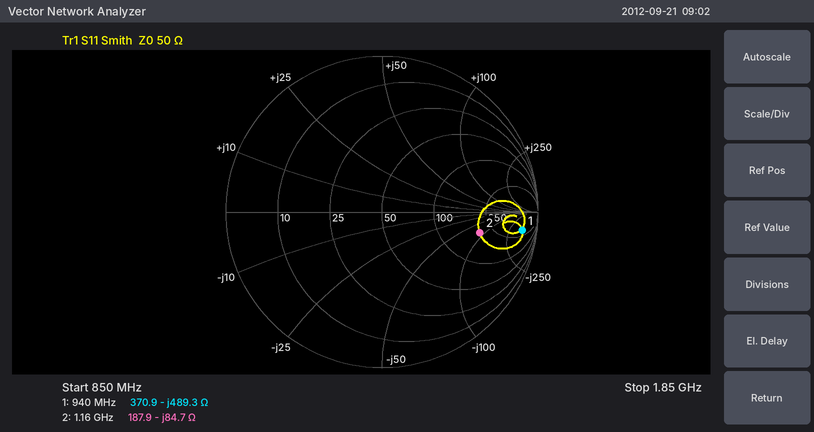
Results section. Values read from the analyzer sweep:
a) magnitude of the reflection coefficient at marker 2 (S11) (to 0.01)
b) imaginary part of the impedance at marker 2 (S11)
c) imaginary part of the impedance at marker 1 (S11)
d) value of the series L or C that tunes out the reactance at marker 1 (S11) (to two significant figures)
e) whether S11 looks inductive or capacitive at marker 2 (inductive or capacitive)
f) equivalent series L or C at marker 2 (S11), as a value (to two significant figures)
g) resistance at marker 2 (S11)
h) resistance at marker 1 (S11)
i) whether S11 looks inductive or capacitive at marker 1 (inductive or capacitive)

0.64
-84.7 Ω
-489.3 Ω
83 nH
capacitive
1.6 pF
187.9 Ω
370.9 Ω
capacitive
